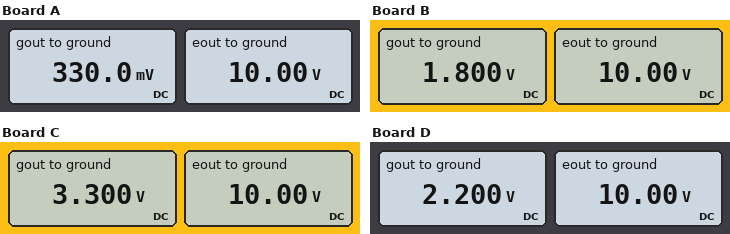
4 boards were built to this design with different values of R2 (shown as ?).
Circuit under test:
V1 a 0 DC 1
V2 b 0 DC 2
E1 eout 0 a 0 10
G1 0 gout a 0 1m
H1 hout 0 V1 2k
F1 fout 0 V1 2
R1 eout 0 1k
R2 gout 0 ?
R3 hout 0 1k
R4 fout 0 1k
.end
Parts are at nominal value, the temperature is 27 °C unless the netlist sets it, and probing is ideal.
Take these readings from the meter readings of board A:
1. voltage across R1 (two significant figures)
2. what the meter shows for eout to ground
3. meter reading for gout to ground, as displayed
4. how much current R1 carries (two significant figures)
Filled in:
10 V
10.00 V
330.0 mV
10 mA
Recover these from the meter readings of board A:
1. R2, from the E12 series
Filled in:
330 Ω
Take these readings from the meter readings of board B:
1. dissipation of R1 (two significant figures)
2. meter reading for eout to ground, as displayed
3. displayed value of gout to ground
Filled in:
100 mW
10.00 V
1.800 V
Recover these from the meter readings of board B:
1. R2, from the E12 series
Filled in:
1.8 kΩ
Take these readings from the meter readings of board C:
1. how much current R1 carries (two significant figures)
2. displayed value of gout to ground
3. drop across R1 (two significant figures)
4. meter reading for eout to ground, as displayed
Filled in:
10 mA
3.300 V
10 V
10.00 V
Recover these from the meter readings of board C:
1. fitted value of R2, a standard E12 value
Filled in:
3.3 kΩ
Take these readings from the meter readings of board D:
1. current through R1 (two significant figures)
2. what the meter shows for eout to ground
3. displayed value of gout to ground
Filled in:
10 mA
10.00 V
2.200 V
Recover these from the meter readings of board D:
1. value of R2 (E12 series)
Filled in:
2.2 kΩ
